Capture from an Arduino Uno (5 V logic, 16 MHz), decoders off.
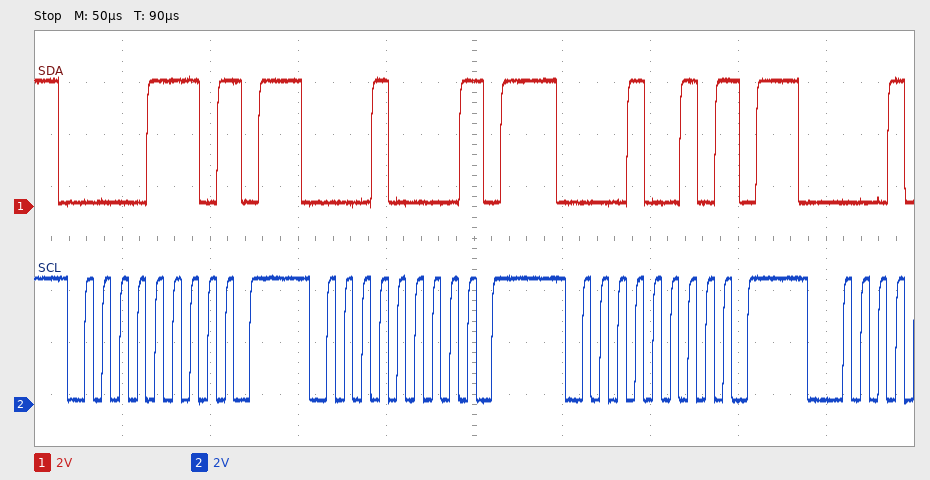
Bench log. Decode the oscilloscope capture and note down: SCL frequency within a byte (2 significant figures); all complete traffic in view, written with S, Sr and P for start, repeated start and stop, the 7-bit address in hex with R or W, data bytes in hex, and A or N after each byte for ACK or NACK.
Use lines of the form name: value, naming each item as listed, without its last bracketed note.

SCL frequency within a byte: 100 kHz
all complete traffic in view, written with S, Sr and P for start, repeated start and stop, the 7-bit address in hex with R or W, data bytes in hex, and A or N after each byte for ACK or NACK: S 07W N P S 08W N P S 09W N P
